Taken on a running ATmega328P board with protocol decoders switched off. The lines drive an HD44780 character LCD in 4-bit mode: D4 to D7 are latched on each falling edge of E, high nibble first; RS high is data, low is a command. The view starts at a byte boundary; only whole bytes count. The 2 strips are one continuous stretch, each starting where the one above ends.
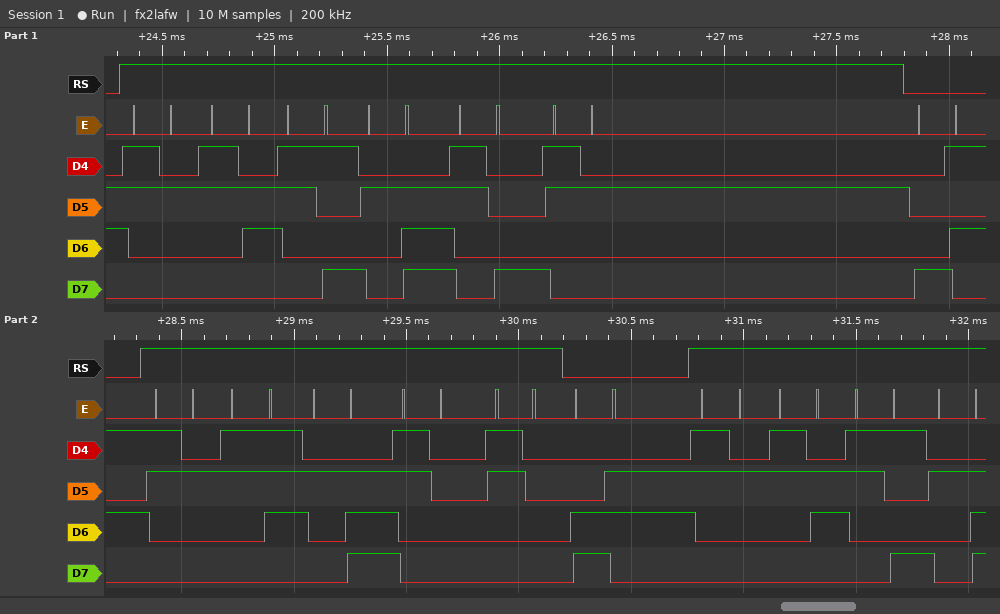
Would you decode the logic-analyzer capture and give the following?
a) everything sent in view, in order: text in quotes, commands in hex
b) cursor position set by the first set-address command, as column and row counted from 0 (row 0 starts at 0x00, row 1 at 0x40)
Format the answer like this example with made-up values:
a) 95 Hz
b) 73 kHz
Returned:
a) "269.82" 0x85 "27.00" 0xC6 "269."
b) column 5, row 0
